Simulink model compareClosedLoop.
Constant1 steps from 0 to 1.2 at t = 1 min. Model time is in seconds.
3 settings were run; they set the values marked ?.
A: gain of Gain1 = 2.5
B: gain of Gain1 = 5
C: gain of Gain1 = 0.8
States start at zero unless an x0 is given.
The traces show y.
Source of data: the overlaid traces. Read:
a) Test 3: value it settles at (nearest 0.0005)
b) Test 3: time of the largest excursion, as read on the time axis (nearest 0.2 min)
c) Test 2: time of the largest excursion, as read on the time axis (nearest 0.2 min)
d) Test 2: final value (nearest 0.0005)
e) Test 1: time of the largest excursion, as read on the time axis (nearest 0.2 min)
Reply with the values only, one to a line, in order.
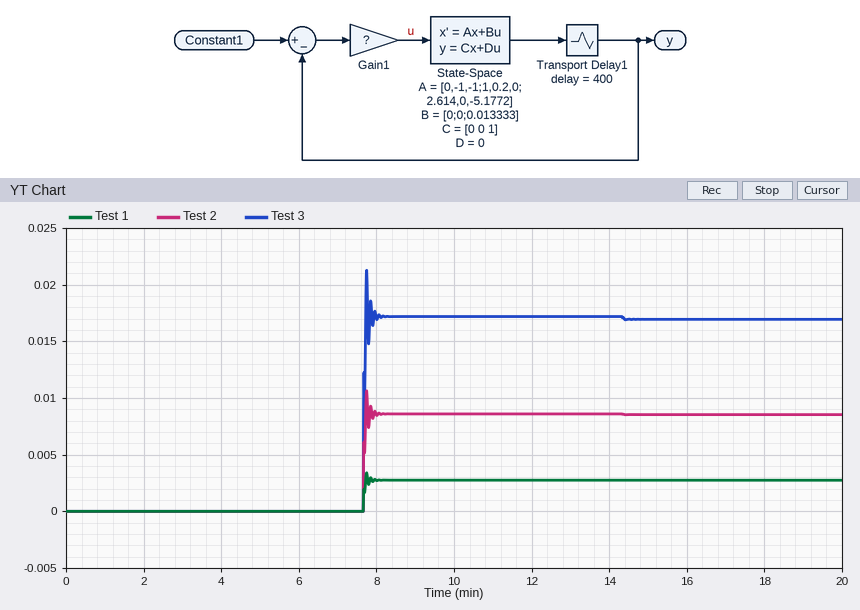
0.0170
7.8 min
7.8 min
0.0085
7.8 min
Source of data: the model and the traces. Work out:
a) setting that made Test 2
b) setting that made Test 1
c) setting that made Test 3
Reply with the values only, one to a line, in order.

A
C
B
